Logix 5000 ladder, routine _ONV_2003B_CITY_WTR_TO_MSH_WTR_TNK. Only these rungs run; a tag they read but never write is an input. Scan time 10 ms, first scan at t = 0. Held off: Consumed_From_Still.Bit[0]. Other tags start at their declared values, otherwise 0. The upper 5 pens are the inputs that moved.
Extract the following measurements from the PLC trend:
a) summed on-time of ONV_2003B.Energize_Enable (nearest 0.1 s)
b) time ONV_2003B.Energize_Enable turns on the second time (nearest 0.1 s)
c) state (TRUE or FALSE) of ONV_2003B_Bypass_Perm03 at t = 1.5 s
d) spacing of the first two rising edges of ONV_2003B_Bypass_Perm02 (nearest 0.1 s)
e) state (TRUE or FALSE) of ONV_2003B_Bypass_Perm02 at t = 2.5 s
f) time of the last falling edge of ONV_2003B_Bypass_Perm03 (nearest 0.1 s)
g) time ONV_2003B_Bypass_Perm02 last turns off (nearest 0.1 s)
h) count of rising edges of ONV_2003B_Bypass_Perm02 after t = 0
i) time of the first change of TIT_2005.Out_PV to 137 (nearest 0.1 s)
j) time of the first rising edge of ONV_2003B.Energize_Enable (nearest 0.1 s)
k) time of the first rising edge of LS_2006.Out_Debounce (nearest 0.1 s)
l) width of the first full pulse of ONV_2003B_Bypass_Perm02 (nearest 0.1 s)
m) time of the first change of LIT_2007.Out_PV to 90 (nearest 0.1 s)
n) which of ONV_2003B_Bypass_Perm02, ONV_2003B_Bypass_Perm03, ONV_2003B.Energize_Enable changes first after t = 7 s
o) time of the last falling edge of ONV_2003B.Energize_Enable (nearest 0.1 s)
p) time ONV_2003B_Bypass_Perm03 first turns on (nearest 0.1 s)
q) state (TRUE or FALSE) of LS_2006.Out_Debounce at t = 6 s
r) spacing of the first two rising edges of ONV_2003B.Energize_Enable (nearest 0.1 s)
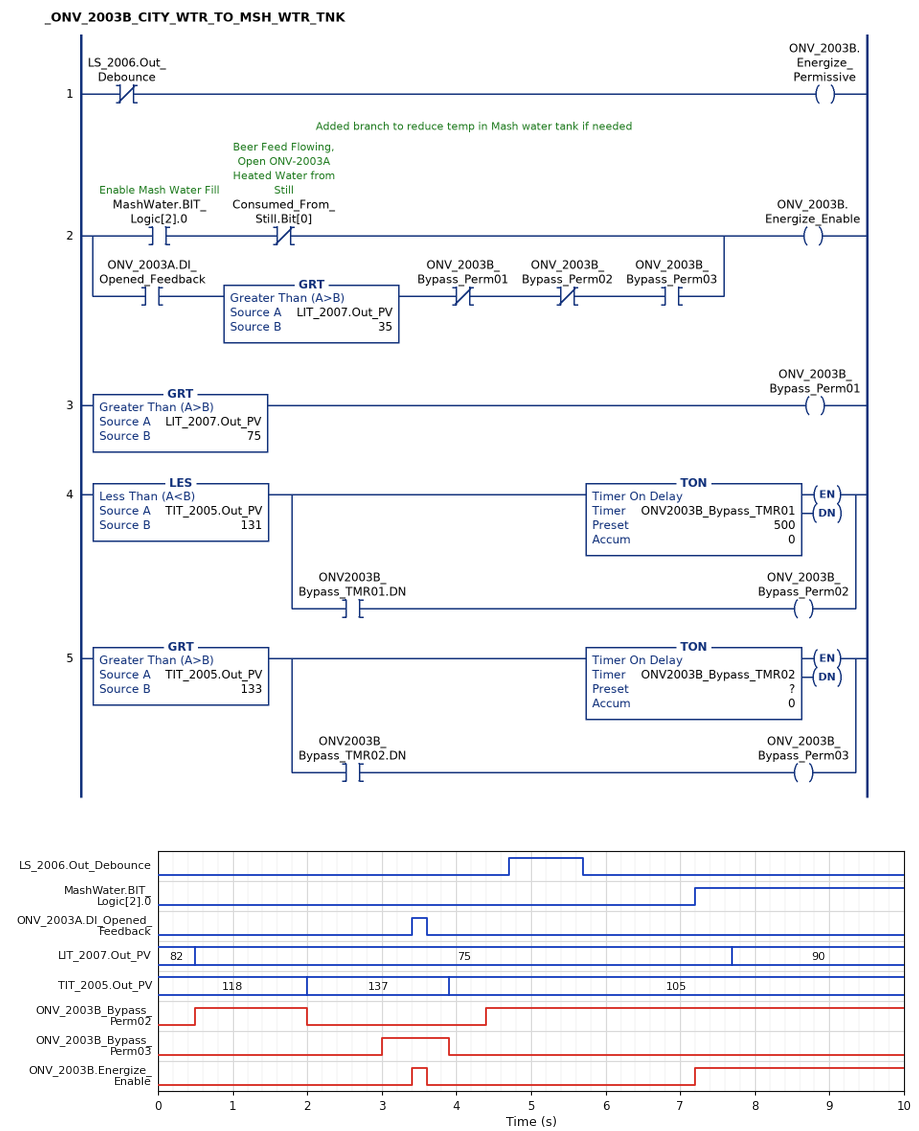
3.0 s
7.2 s
FALSE
3.9 s
FALSE
3.9 s
2.0 s
2
2.0 s
3.4 s
4.7 s
1.5 s
7.7 s
ONV_2003B.Energize_Enable
3.6 s
3.0 s
FALSE
3.8 s
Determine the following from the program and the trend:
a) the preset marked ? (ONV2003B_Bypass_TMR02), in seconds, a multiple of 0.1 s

1.0 s
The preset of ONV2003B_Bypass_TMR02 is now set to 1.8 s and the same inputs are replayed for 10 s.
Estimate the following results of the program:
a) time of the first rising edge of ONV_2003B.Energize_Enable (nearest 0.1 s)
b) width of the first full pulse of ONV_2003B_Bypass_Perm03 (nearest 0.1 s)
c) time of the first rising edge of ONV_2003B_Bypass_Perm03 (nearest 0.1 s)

7.2 s
0.1 s
3.8 s
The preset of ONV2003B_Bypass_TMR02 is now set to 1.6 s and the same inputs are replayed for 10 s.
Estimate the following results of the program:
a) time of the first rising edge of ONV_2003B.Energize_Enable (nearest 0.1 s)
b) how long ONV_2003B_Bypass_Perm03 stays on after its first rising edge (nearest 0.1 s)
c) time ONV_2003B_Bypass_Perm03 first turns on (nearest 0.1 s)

7.2 s
0.3 s
3.6 s
